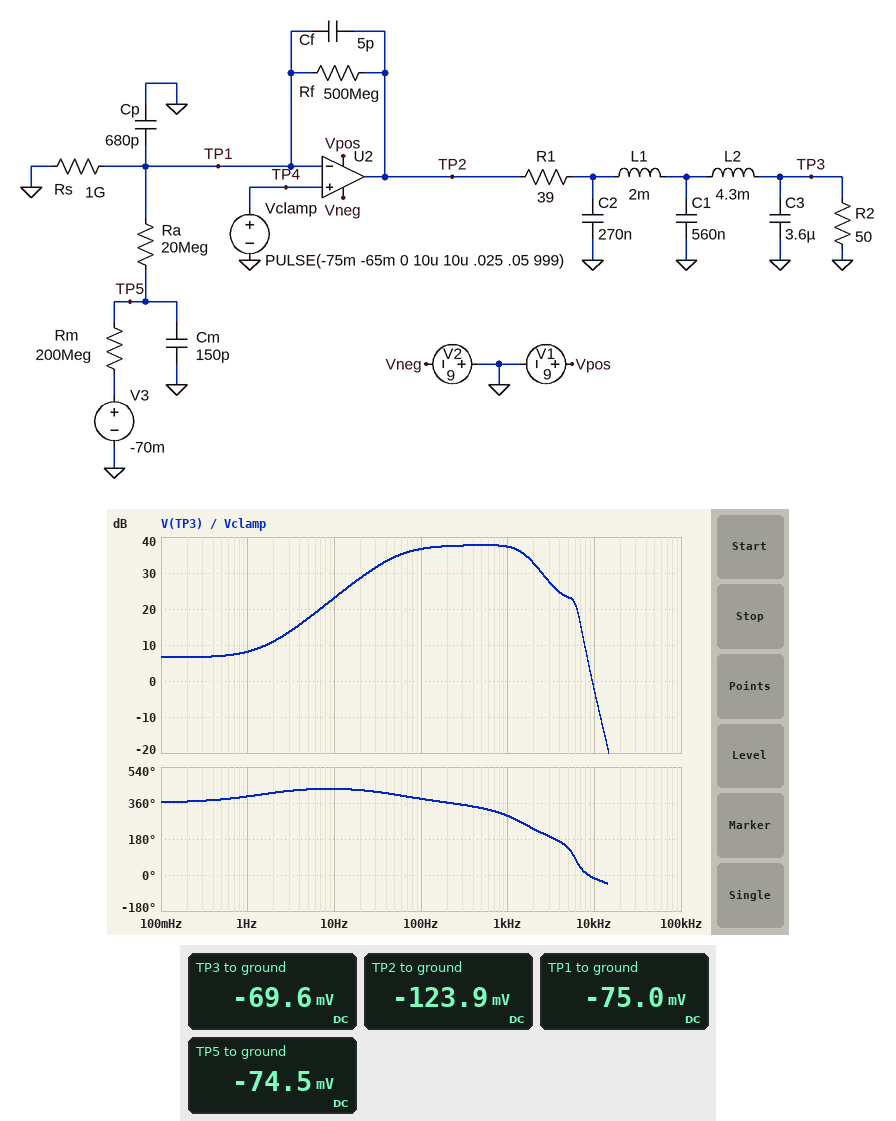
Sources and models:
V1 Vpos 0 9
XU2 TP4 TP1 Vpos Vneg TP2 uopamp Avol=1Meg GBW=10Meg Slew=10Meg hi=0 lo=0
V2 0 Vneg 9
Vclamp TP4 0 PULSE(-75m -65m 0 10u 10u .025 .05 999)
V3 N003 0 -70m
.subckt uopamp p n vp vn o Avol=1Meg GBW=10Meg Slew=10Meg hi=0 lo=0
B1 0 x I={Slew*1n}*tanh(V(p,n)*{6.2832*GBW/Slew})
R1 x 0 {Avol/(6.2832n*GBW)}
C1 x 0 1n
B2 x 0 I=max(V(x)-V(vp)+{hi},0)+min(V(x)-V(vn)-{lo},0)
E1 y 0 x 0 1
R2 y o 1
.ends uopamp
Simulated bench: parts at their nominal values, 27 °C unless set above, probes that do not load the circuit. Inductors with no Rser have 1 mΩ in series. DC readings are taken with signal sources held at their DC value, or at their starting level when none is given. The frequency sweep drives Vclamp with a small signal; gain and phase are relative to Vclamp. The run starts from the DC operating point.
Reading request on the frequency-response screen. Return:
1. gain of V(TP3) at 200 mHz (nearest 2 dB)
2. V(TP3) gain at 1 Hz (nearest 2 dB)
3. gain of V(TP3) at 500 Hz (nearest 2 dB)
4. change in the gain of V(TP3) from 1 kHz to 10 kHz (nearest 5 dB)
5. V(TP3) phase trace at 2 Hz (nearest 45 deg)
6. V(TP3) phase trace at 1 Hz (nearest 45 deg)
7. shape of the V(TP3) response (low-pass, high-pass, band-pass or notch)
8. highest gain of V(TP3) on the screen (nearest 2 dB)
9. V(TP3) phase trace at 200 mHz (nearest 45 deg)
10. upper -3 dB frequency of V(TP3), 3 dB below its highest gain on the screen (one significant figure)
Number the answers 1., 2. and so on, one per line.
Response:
1. 6 dB
2. 8 dB
3. 38 dB
4. -40 dB
5. 405 deg
6. 405 deg
7. band-pass
8. 38 dB
9. 360 deg
10. 2 kHz
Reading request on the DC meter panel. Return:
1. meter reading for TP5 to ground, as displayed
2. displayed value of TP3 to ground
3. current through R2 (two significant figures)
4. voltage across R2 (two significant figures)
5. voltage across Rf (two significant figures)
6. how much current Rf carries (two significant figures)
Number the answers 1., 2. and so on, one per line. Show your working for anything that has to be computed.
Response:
1. -74.5 mV
2. -69.6 mV
3. (0 V - (-69.6 mV)) / 50 Ω = 1.4 mA
4. 0 V - (-69.6 mV) = 70 mV
5. -75 mV - (-123.9 mV) = 49 mV
6. (-75 mV - (-123.9 mV)) / 500 MΩ = 98 pA
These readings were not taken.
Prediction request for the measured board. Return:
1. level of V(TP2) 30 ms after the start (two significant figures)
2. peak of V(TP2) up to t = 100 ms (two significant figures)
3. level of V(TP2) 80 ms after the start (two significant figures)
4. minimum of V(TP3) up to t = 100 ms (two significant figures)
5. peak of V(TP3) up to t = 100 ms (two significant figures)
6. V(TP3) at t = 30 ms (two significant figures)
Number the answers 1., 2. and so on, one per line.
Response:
1. -370 mV
2. 1.2 V
3. -370 mV
4. -800 mV
5. 680 mV
6. -220 mV
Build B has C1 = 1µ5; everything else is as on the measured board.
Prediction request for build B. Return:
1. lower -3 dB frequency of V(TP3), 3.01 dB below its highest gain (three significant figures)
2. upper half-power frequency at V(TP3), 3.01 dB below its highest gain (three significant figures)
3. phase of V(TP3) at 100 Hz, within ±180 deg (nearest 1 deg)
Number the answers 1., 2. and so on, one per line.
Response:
1. 52.3 Hz
2. 1.98 kHz
3. 20 deg
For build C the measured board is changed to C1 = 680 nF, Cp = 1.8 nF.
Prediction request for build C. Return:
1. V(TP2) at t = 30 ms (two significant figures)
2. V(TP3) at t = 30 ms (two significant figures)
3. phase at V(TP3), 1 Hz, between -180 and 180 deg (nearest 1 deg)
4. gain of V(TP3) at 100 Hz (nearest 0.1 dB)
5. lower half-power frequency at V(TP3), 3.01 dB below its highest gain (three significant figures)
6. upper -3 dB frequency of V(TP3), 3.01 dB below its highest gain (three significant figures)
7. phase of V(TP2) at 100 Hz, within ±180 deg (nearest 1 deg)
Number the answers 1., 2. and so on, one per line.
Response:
1. -680 mV
2. -400 mV
3. 57 deg
4. 44.8 dB
5. 59.4 Hz
6. 1.67 kHz
7. 30 deg
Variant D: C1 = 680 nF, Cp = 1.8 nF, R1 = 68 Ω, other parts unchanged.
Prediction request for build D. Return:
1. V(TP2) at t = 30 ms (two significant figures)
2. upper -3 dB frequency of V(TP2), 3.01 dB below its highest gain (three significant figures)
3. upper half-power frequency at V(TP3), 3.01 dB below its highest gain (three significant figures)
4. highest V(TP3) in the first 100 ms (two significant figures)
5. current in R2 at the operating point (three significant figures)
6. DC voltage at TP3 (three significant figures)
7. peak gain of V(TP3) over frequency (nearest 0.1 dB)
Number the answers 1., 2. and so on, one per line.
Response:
1. -680 mV
2. 27.5 kHz
3. 1.88 kHz
4. 1.3 V
5. 1.05 mA
6. -52.5 mV
7. 43.4 dB
